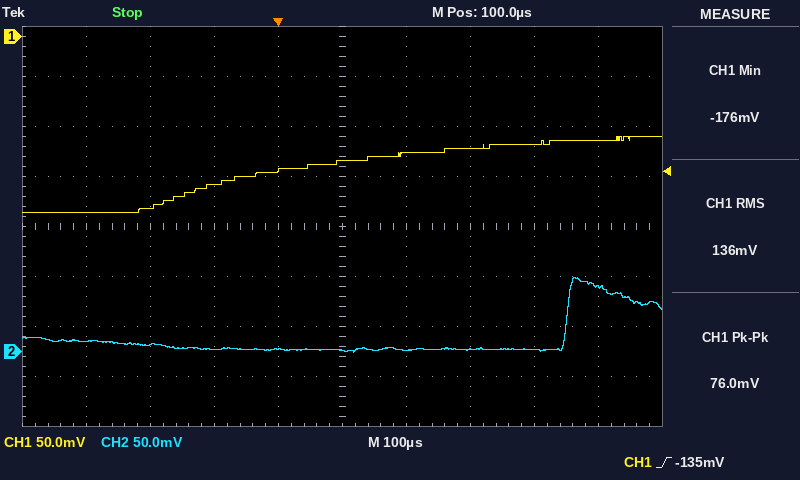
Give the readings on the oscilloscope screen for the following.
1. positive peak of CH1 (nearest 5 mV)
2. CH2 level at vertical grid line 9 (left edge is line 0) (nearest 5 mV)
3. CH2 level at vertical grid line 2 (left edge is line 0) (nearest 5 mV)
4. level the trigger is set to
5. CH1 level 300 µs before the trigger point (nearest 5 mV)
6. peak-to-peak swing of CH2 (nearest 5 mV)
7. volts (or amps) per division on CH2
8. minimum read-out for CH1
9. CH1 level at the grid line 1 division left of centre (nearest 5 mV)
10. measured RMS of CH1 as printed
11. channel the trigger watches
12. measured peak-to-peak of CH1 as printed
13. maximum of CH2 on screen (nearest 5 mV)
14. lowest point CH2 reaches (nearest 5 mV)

-100 mV
65 mV
5 mV
-135 mV
-175 mV
75 mV
50 mV
-176 mV
-135 mV
136 mV
CH1
76.0 mV
75 mV
0 mV
